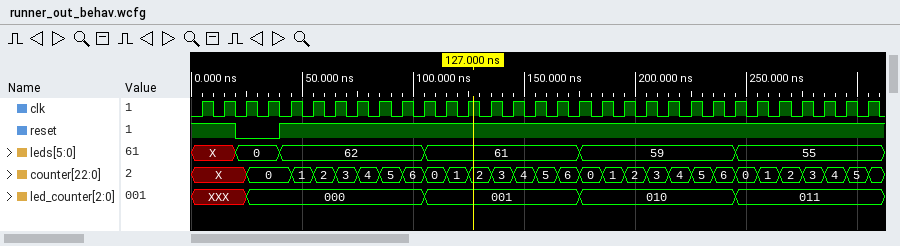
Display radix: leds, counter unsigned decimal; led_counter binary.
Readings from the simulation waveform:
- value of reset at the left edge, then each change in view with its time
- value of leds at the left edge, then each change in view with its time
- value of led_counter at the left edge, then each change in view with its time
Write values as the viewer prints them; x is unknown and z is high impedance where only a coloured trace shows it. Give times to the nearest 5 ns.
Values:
1, 0 at 20 ns, 1 at 40 ns
X, 0 at 20 ns, 62 at 40 ns, 61 at 105 ns, 59 at 175 ns, 55 at 245 ns
XXX, 000 at 25 ns, 001 at 105 ns, 010 at 175 ns, 011 at 245 ns
